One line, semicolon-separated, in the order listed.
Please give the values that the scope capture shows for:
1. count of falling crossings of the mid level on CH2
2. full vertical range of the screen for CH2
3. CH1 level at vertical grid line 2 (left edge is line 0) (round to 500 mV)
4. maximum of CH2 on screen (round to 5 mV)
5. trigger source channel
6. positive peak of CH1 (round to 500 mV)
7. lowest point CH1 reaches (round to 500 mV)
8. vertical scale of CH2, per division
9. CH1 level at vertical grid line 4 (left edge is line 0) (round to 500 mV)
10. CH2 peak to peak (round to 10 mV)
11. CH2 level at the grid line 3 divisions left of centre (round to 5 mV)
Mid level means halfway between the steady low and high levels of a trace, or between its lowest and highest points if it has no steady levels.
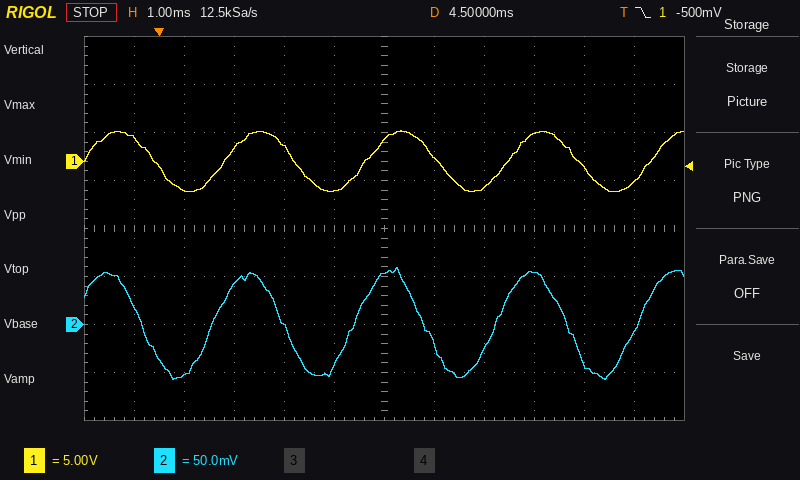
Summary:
4; 400 mV; -3.0 V; 60 mV; CH1; 3.0 V; -3.0 V; 50 mV; 1.5 V; 120 mV; 40 mV
